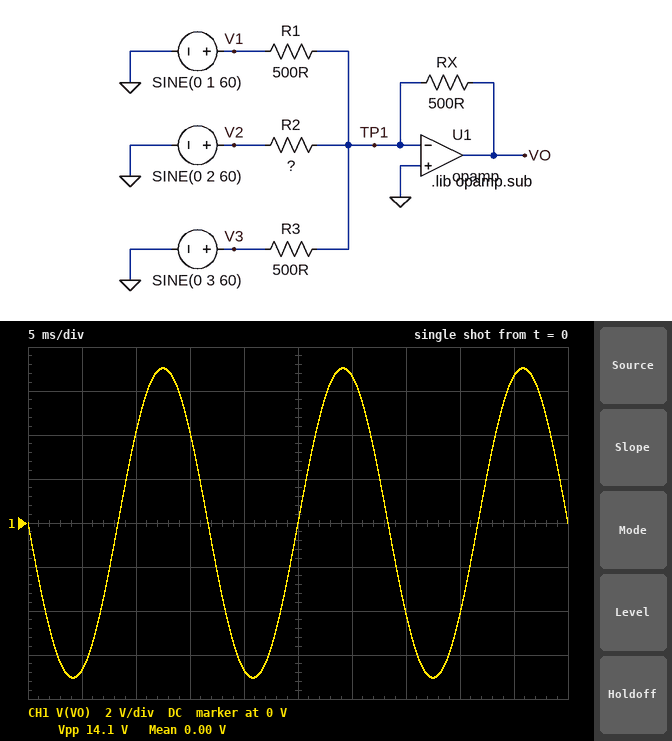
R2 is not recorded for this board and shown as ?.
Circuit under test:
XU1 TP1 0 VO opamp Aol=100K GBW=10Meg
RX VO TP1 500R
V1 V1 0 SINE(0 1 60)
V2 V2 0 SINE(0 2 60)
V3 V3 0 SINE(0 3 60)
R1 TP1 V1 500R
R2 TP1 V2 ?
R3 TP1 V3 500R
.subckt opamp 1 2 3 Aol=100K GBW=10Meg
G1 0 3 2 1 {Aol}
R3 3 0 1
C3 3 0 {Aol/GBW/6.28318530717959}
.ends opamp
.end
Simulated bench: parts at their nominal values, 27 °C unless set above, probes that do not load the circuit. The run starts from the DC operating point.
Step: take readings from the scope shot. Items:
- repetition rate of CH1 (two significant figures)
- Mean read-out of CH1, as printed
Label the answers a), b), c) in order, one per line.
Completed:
a) 60 Hz
b) 0.00 V
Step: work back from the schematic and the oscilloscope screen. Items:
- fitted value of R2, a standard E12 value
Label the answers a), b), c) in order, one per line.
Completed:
a) 330 Ω
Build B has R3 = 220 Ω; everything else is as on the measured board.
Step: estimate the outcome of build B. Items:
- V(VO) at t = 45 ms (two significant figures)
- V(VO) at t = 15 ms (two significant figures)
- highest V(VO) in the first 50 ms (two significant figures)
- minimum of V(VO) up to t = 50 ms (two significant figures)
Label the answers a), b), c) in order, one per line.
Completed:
a) 10 V
b) 6.4 V
c) 11 V
d) -11 V
